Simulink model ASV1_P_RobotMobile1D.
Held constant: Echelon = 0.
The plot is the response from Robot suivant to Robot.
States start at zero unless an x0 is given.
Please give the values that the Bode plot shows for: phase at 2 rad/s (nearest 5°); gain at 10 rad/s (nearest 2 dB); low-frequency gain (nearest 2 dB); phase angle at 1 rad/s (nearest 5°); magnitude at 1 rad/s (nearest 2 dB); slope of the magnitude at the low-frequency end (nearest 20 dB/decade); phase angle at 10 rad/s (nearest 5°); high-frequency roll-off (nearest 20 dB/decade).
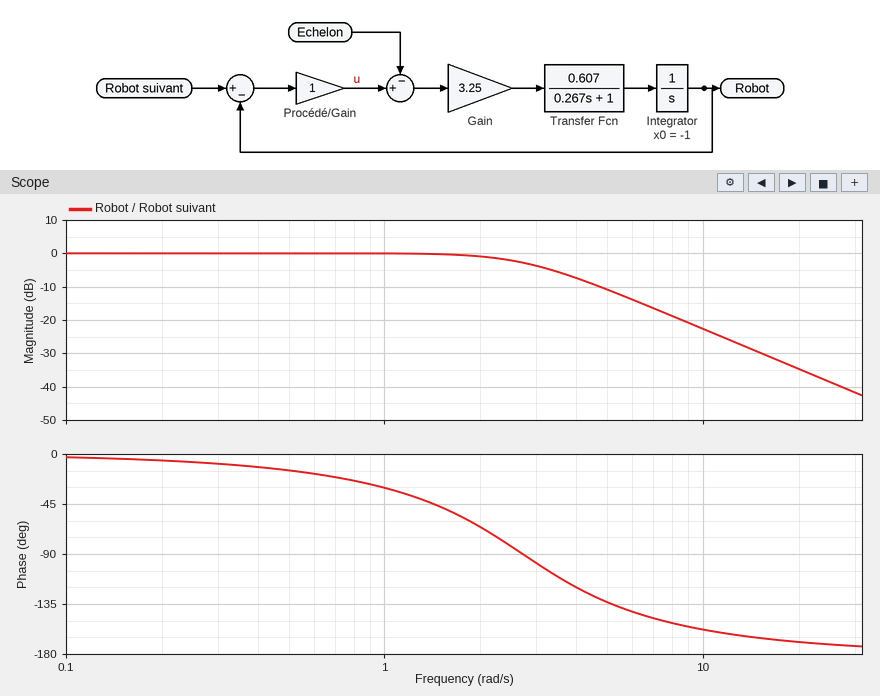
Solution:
-65°
-22 dB
0 dB
-30°
0 dB
0 dB/decade
-160°
-40 dB/decade
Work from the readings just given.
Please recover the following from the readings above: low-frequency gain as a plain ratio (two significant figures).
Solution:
1.0
